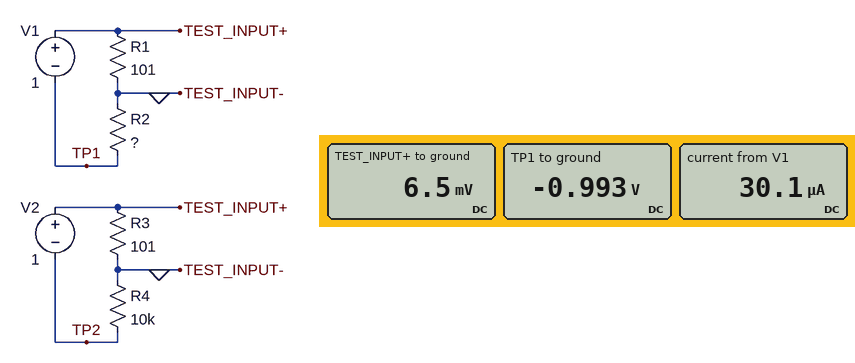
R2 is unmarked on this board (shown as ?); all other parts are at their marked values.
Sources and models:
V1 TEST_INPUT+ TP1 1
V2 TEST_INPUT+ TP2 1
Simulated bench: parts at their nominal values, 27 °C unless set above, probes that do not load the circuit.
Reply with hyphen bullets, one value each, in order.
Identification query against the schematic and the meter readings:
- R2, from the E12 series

- 33 kΩ
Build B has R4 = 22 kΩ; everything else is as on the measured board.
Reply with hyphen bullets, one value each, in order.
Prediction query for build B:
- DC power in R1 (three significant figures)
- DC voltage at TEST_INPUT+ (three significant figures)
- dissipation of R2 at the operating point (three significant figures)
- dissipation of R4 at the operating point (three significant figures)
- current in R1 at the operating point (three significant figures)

- 144 nW
- 3.81 mV
- 30.1 µW
- 45.1 µW
- 37.7 µA
